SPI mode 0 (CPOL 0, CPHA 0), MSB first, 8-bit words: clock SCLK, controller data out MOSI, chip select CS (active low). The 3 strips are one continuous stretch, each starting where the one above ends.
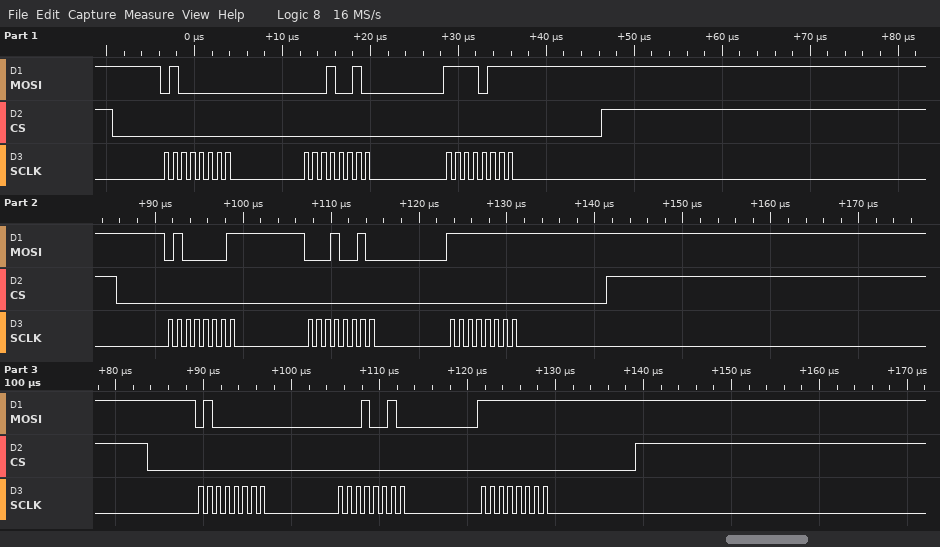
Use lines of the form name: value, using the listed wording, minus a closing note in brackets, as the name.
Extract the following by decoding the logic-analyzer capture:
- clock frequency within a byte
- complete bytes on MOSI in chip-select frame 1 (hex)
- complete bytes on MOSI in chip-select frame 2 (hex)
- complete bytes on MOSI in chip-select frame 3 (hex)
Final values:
clock frequency within a byte: 1 MHz
complete bytes on MOSI in chip-select frame 1: 40 12 F7
complete bytes on MOSI in chip-select frame 2: 41 12 FF
complete bytes on MOSI in chip-select frame 3: 40 12 FF
